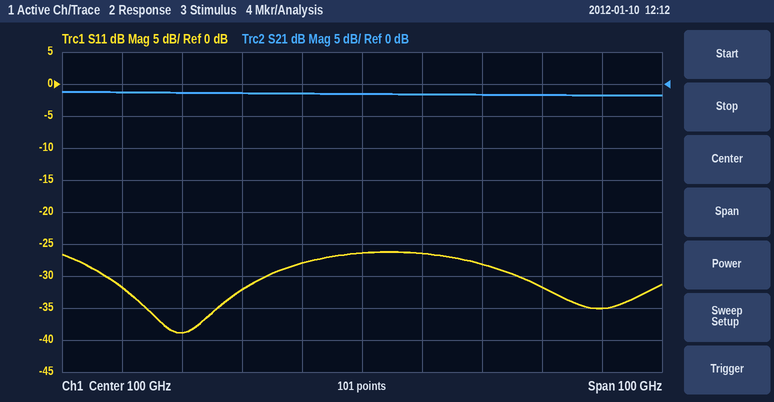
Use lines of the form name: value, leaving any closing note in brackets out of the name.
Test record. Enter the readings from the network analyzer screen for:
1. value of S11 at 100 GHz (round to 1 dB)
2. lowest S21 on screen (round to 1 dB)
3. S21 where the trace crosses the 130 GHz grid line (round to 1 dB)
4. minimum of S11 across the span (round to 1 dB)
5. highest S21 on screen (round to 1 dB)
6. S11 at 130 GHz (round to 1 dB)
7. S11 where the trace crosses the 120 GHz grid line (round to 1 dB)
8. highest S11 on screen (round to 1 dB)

value of S11 at 100 GHz: -26 dB
lowest S21 on screen: -2 dB
S21 where the trace crosses the 130 GHz grid line: -2 dB
minimum of S11 across the span: -39 dB
highest S21 on screen: -1 dB
S11 at 130 GHz: -32 dB
S11 where the trace crosses the 120 GHz grid line: -28 dB
highest S11 on screen: -26 dB
